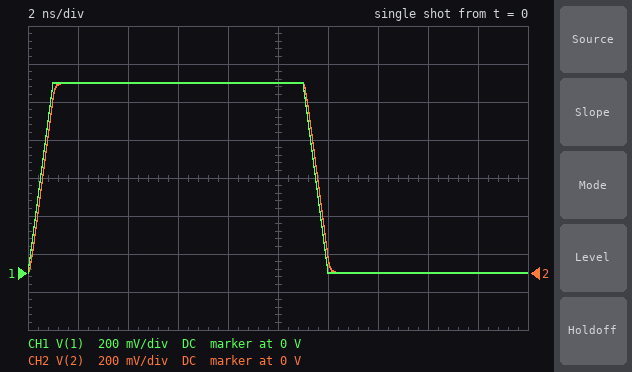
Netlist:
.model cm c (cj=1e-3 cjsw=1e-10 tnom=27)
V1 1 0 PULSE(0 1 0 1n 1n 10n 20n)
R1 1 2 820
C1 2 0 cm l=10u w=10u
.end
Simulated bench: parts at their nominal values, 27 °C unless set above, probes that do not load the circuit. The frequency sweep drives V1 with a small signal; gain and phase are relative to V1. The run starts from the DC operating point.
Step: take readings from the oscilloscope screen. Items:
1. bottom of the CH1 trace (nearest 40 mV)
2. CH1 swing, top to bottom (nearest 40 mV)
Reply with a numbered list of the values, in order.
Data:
1. 0 V
2. 1.00 V
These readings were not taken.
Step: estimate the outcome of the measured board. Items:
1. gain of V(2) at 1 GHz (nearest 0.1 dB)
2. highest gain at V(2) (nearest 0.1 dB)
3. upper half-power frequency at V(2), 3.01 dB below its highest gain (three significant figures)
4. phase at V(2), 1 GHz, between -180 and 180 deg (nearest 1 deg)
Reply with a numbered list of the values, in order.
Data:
1. -1.1 dB
2. 0 dB
3. 1.87 GHz
4. -28 deg
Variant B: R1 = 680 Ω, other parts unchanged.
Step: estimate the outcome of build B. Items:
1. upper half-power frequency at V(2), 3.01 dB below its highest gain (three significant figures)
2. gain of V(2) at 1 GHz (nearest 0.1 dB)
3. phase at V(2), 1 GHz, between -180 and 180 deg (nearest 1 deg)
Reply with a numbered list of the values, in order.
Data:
1. 2.25 GHz
2. -0.8 dB
3. -24 deg
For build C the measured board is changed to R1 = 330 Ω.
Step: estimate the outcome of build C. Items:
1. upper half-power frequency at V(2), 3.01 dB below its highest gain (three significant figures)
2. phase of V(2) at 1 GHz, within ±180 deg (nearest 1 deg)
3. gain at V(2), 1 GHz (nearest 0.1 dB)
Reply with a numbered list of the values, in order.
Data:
1. 4.64 GHz
2. -12 deg
3. -0.2 dB
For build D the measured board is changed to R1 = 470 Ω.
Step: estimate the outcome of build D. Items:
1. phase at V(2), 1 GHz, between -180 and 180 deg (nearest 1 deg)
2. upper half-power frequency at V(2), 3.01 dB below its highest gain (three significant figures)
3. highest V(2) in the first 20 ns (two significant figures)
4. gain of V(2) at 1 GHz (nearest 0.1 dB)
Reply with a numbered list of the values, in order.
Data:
1. -17 deg
2. 3.26 GHz
3. 1.0 V
4. -0.4 dB
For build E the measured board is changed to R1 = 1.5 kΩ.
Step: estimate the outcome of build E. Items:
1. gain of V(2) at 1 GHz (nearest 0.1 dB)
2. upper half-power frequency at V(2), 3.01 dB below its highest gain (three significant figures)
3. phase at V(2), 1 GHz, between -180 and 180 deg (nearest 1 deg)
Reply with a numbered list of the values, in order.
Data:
1. -2.9 dB
2. 1.02 GHz
3. -44 deg
